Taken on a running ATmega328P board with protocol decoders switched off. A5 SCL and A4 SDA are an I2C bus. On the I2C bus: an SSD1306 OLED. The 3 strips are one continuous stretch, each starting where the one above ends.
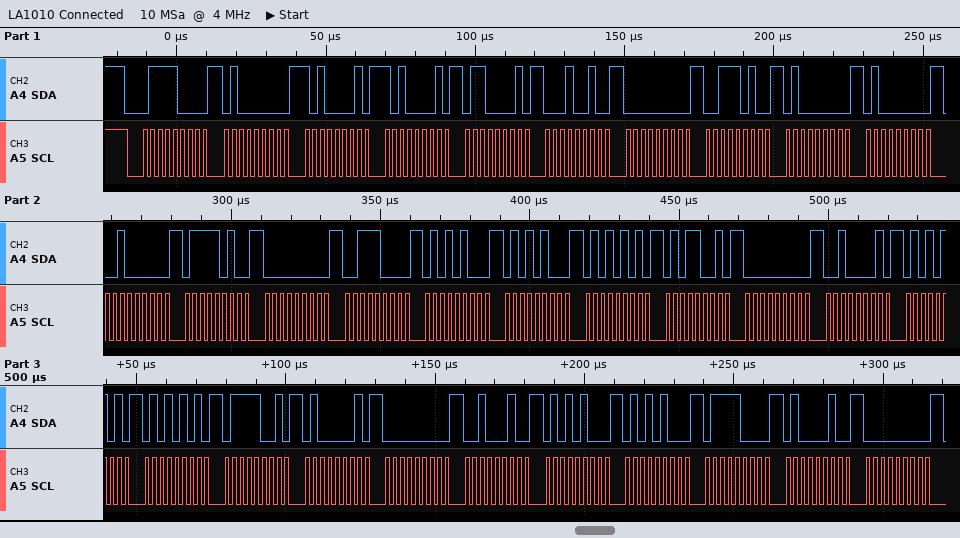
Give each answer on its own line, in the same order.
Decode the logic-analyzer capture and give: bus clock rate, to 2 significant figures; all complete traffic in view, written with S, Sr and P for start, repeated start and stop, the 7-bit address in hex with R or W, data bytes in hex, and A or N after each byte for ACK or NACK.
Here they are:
400 kHz
S 3CW A 40 A A1 A A1 A 61 A 12 A 00 A 3A A 40 A 40 A 20 A 7A A 00 A 38 A 54 A 54 A 55 A 59 A 00 A 21 A 55 A 55 A 79 A 41 A 00 A 22 A 54 A 54 A 78 A 42 A 00 A
